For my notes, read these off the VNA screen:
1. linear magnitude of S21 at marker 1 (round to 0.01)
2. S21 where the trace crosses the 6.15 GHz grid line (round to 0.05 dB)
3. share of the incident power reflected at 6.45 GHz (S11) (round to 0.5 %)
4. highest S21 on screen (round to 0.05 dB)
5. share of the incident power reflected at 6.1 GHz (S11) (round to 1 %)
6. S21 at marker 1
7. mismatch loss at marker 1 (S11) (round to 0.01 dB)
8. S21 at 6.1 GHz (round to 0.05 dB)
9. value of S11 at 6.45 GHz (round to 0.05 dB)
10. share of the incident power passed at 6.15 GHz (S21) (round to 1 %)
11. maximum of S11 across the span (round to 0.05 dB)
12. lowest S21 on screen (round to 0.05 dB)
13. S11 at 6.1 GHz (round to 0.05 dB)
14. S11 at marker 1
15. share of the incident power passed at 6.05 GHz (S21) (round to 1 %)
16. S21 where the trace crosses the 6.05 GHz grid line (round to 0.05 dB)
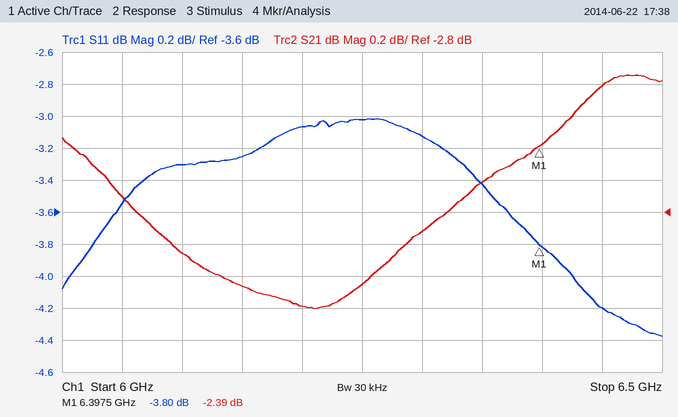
0.76
-3.25 dB
38.0 %
-1.95 dB
47 %
-2.39 dB
2.34 dB
-3.05 dB
-4.20 dB
47 %
-3.00 dB
-3.40 dB
-3.30 dB
-3.80 dB
54 %
-2.70 dB
